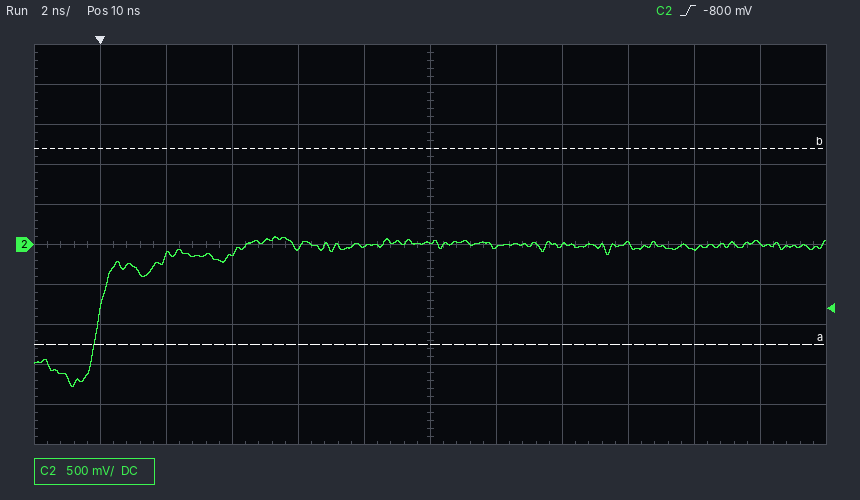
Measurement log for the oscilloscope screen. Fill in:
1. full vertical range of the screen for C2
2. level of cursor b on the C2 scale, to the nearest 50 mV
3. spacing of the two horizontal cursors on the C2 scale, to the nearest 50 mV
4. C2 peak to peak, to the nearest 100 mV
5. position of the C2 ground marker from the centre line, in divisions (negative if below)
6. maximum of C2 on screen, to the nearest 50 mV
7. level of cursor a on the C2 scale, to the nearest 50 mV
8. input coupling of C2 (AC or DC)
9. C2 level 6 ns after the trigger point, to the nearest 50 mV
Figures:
5 V
1.20 V
2.45 V
1.90 V
0.0 div
100 mV
-1.25 V
DC
-50 mV
